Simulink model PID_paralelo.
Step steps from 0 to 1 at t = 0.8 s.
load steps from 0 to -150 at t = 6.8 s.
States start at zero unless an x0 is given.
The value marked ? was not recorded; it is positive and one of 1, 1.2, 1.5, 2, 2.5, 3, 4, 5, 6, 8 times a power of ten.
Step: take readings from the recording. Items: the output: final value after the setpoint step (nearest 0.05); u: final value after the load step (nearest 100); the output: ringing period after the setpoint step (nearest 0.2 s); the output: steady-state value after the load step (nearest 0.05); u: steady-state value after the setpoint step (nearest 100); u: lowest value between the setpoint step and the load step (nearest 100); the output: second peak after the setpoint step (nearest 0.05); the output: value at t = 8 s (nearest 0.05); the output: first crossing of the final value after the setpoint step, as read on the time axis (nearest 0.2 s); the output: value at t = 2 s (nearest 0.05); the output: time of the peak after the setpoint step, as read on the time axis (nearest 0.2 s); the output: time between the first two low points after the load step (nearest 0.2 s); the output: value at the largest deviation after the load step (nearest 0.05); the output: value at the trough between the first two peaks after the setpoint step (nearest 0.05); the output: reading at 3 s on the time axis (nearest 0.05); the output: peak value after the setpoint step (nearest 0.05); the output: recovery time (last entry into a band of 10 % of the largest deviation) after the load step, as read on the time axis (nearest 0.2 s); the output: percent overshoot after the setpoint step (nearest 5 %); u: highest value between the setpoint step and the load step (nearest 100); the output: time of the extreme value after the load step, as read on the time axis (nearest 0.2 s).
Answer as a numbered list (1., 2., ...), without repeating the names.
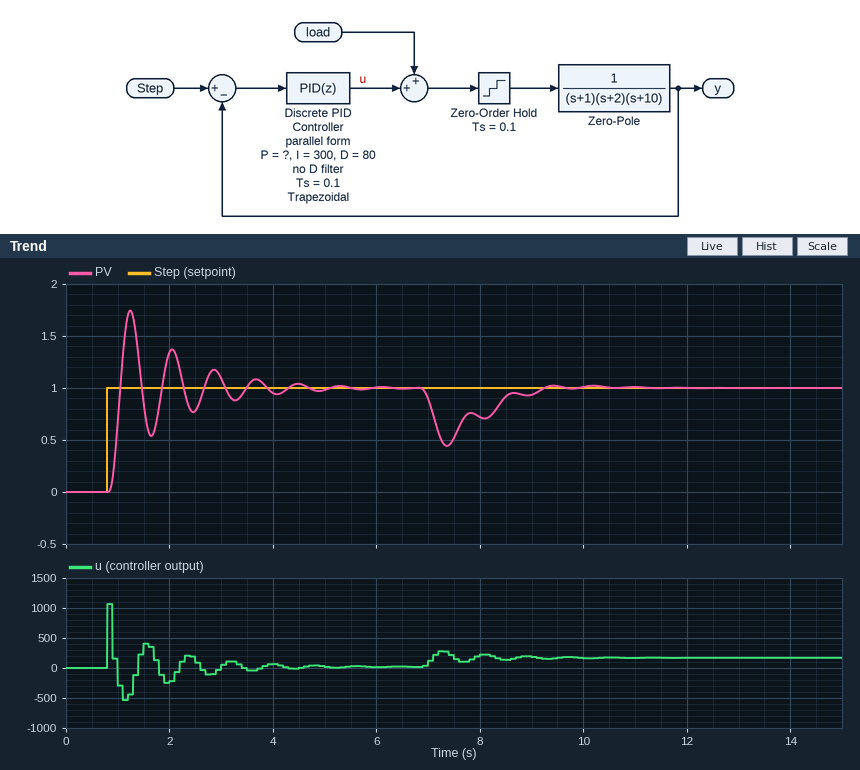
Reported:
1. 1.00
2. 200
3. 0.8 s
4. 1.00
5. 0
6. -500
7. 1.35
8. 0.70
9. 1.0 s
10. 1.35
11. 1.2 s
12. 0.8 s
13. 0.45
14. 0.55
15. 1.10
16. 1.75
17. 9.0 s
18. 75 %
19. 1100
20. 7.4 s
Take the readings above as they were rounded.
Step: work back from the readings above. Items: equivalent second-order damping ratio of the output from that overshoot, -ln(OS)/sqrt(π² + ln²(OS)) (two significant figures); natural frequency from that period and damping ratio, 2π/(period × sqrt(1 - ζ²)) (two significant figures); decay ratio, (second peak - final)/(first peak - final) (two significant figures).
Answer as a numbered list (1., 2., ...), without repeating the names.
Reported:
1. 0.091
2. 7.9 rad/s
3. 0.47
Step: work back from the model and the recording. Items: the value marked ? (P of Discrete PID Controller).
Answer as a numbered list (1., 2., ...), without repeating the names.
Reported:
1. 250
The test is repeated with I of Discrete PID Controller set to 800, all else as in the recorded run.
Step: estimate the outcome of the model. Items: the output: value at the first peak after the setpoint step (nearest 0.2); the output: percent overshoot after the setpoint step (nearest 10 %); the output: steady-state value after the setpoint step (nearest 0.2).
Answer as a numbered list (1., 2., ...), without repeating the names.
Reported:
1. 2.0
2. 100 %
3. 1.0
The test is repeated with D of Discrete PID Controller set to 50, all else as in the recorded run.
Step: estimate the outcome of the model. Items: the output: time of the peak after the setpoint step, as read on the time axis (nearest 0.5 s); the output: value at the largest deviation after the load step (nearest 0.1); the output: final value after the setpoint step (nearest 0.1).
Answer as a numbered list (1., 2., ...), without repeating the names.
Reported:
1. 1.5 s
2. 0.3
3. 1.0
